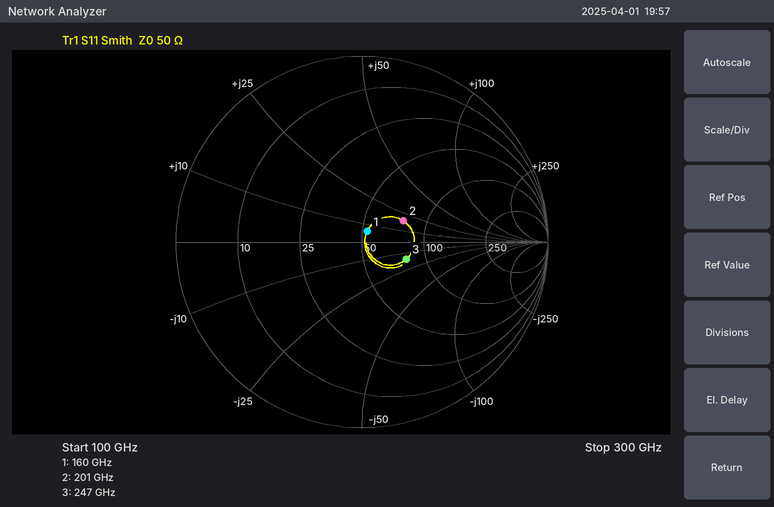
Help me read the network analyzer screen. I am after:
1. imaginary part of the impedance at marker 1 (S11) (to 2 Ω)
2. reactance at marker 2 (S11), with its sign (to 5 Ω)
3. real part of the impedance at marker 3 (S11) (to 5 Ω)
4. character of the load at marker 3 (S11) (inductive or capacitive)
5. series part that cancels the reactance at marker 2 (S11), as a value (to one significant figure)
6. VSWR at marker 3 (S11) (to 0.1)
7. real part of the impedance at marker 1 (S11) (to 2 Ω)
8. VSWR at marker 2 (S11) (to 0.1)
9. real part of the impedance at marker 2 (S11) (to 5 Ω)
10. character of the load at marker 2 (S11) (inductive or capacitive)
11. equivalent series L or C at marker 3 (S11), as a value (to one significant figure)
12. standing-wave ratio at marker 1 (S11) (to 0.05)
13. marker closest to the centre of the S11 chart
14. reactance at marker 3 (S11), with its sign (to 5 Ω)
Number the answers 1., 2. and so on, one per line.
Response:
1. +6 Ω
2. +20 Ω
3. 80 Ω
4. capacitive
5. 40 fF
6. 1.7
7. 52 Ω
8. 1.7
9. 75 Ω
10. inductive
11. 40 fF
12. 1.15
13. marker 1
14. -15 Ω
